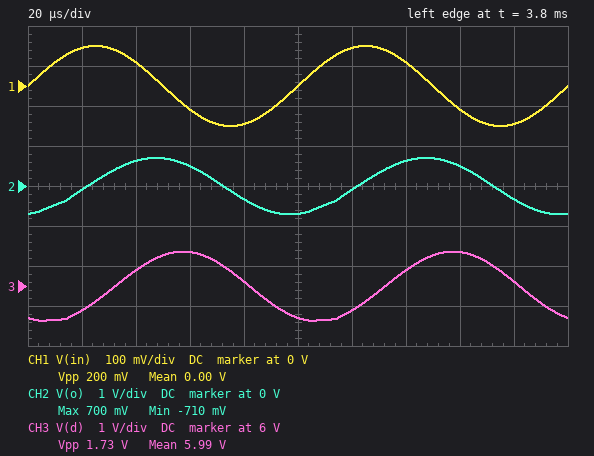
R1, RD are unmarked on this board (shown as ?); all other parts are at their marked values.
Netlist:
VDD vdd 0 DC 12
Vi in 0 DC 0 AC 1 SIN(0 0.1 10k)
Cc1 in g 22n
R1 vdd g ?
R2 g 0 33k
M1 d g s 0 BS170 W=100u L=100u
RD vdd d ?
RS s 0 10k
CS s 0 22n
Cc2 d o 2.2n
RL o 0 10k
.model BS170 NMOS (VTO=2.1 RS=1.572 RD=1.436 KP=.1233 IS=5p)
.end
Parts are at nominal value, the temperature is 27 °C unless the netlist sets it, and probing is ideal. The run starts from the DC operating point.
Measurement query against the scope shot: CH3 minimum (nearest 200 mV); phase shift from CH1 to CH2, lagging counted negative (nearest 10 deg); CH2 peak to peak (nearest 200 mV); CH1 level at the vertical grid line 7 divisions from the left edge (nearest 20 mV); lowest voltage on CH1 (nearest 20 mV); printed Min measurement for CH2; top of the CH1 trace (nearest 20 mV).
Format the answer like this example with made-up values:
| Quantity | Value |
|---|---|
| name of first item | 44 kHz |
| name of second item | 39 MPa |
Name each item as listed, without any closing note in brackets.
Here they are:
| Quantity | Value |
|---|---|
| CH3 minimum | 5.2 V |
| phase shift from CH1 to CH2, lagging counted negative | -80 deg |
| CH2 peak to peak | 1.4 V |
| CH1 level at the vertical grid line 7 divisions from the left edge | 60 mV |
| lowest voltage on CH1 | -100 mV |
| printed Min measurement for CH2 | -710 mV |
| top of the CH1 trace | 100 mV |
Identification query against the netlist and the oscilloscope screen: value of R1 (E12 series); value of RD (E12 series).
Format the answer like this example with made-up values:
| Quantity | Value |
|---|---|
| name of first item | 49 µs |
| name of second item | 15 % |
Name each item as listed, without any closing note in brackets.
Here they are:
| Quantity | Value |
|---|---|
| value of R1 | 22 kΩ |
| value of RD | 12 kΩ |
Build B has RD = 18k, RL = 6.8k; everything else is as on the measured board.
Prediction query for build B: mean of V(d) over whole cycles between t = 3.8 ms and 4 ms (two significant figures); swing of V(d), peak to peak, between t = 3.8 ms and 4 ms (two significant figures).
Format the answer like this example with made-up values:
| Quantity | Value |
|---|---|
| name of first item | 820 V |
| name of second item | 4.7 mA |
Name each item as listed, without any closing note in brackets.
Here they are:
| Quantity | Value |
|---|---|
| mean of V(d) over whole cycles between t = 3.8 ms and 4 ms | 4.3 V |
| swing of V(d), peak to peak, between t = 3.8 ms and 4 ms | 1.0 mV |
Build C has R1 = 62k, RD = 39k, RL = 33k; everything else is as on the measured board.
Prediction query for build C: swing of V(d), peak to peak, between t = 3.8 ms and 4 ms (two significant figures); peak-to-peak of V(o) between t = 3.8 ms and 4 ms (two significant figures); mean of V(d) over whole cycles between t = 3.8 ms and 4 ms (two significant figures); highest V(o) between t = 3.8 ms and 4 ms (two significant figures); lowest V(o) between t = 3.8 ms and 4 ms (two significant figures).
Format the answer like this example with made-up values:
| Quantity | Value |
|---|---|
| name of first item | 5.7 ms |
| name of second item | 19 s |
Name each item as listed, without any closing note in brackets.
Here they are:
| Quantity | Value |
|---|---|
| swing of V(d), peak to peak, between t = 3.8 ms and 4 ms | 4.5 V |
| peak-to-peak of V(o) between t = 3.8 ms and 4 ms | 4.6 V |
| mean of V(d) over whole cycles between t = 3.8 ms and 4 ms | 4.2 V |
| highest V(o) between t = 3.8 ms and 4 ms | 2.3 V |
| lowest V(o) between t = 3.8 ms and 4 ms | -2.3 V |
